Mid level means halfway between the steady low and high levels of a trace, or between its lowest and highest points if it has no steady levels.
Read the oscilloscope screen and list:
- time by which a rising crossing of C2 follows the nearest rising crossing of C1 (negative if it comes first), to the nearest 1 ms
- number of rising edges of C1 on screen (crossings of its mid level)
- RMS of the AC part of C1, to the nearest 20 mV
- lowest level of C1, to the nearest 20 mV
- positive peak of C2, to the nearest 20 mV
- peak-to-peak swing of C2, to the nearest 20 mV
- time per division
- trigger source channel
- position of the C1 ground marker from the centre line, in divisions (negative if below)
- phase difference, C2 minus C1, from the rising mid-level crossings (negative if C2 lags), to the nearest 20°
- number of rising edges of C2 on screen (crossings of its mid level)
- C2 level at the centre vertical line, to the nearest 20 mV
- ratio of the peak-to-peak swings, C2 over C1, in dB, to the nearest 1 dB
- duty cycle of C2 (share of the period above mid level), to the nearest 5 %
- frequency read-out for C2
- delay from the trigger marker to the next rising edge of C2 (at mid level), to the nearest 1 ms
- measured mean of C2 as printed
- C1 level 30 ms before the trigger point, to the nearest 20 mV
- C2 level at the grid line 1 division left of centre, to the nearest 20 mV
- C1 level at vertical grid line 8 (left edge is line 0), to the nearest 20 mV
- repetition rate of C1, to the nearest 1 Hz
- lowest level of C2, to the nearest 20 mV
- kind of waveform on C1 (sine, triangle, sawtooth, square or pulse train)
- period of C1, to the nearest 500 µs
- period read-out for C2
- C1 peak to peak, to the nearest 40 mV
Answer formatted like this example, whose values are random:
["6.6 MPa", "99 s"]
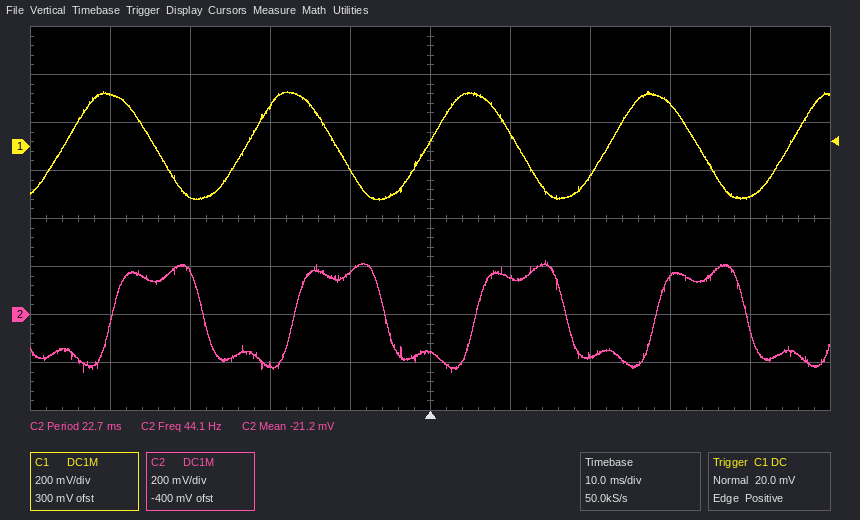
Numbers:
["+6 ms", "5", "160 mV", "-220 mV", "220 mV", "460 mV", "10 ms", "C1", "+1.5 div", "-100°", "4", "-160 mV", "0 dB", "50 %", "44.1 Hz", "6 ms", "-21.2 mV", "-200 mV", "180 mV", "180 mV", "44 Hz", "-240 mV", "sine", "22.5 ms", "22.7 ms", "440 mV"]
